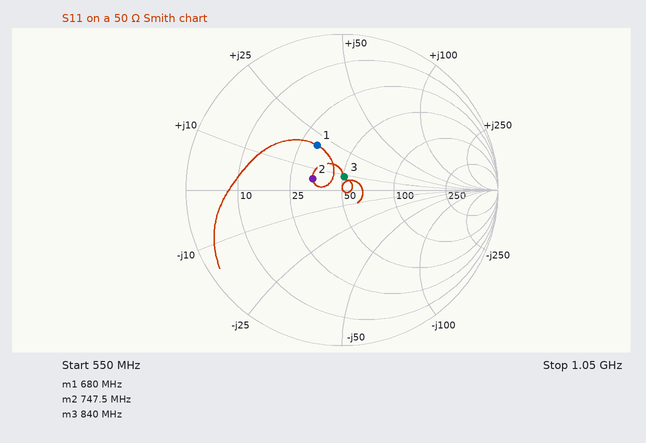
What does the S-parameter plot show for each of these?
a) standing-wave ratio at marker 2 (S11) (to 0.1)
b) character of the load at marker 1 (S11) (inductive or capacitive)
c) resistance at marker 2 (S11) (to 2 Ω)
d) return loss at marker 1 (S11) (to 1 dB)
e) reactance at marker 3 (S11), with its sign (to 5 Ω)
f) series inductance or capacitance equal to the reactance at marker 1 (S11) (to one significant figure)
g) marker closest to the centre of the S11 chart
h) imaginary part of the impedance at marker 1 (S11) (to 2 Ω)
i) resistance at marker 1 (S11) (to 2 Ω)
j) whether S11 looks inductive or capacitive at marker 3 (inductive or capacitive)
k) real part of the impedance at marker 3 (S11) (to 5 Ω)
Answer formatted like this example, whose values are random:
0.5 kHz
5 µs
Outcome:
1.5
inductive
34 Ω
10 dB
+10 Ω
5 nH
marker 3
+20 Ω
32 Ω
inductive
50 Ω
